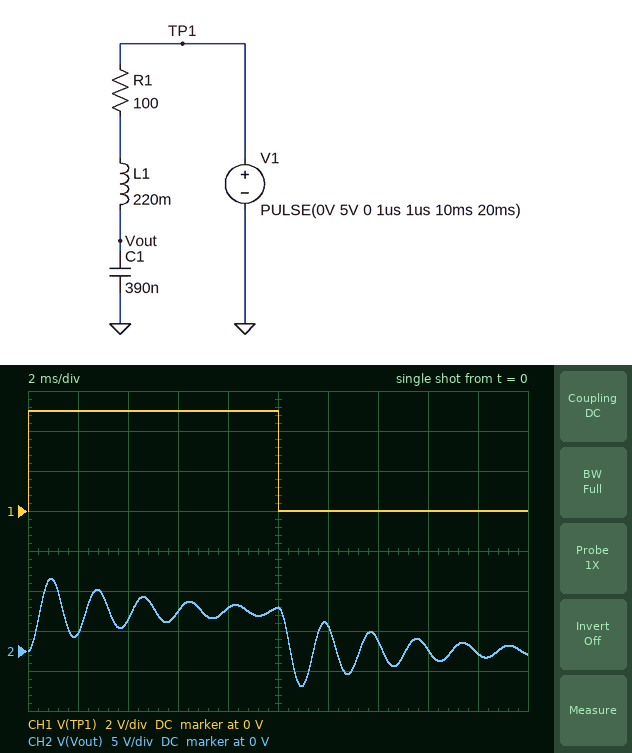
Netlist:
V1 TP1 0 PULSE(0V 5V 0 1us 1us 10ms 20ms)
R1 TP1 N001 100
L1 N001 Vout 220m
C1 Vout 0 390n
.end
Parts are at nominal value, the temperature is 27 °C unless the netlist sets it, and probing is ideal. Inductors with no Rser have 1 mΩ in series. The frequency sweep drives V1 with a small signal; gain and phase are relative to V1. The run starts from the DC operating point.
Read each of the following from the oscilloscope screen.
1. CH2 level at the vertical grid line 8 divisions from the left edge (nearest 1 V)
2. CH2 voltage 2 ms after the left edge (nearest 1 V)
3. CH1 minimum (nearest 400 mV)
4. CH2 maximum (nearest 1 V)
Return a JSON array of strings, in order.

["0 V", "2 V", "0 V", "9 V"]
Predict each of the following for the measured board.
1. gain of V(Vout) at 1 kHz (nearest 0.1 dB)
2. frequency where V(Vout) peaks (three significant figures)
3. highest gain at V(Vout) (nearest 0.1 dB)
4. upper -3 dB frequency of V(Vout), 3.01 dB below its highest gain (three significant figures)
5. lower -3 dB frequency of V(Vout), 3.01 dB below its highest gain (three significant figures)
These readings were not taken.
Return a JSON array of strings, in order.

["-7.6 dB", "541 Hz", "17.5 dB", "576 Hz", "503 Hz"]
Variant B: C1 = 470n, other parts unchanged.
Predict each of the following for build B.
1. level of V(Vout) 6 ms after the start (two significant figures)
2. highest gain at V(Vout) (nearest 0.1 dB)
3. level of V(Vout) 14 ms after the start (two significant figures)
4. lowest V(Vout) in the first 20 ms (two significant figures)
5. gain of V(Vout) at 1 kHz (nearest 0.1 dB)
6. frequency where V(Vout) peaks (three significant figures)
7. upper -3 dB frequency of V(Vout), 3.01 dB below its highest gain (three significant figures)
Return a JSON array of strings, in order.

["3.8 V", "16.7 dB", "1.8 V", "-3.6 V", "-9.8 dB", "492 Hz", "527 Hz"]
